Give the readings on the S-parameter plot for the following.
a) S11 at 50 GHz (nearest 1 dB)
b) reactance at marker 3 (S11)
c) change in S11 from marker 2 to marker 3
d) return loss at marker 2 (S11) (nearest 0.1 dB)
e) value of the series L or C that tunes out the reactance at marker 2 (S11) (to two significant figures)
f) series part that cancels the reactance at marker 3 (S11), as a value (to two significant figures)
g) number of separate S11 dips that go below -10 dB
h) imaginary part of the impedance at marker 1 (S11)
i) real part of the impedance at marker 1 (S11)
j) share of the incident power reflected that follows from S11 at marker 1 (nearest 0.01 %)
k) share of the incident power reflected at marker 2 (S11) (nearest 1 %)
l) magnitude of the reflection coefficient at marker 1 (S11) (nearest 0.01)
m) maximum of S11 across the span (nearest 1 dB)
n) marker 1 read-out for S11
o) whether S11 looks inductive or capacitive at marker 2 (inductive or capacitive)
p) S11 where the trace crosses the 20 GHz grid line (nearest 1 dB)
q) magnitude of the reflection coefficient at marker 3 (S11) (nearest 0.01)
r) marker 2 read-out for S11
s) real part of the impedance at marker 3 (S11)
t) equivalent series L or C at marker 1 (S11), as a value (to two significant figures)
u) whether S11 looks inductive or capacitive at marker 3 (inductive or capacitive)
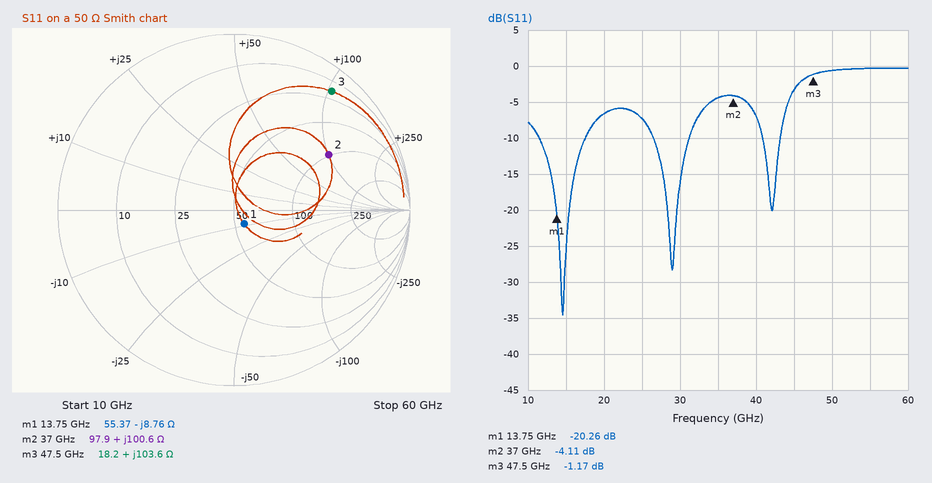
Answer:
-1 dB
+103.6 Ω
2.94 dB
4.1 dB
43 fF
32 fF
3
-8.76 Ω
55.37 Ω
0.94 %
39 %
0.10
0 dB
-20.26 dB
inductive
-7 dB
0.87
-4.11 dB
18.2 Ω
1.3 pF
inductive
